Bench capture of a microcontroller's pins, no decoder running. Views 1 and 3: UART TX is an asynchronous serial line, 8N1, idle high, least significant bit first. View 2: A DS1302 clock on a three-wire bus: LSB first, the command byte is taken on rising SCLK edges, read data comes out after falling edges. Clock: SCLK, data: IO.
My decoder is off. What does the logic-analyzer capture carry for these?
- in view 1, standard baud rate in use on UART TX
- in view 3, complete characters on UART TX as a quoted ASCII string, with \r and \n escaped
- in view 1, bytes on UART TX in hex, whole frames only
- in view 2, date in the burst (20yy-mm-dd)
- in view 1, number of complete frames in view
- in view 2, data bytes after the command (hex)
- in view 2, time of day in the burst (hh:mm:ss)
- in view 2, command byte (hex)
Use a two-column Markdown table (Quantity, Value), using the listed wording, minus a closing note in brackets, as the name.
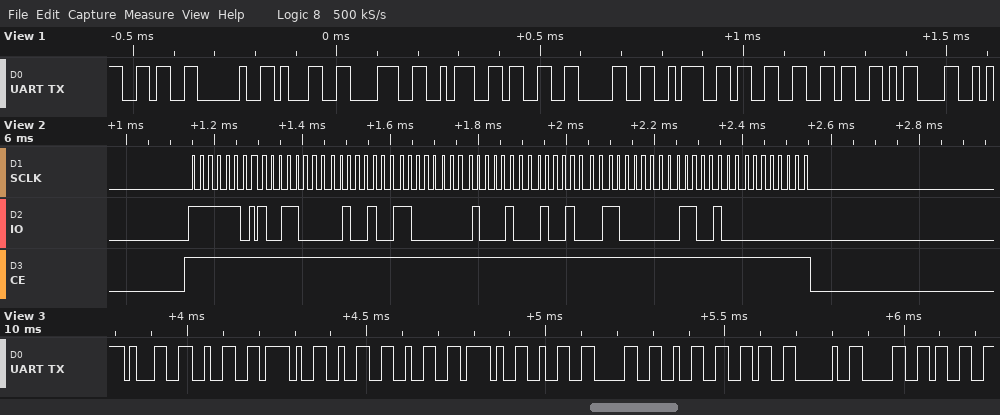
| Quantity | Value |
|---|---|
| in view 1, standard baud rate in use on UART TX | 57600 baud |
| in view 3, complete characters on UART TX as a quoted ASCII string, with \r and \n escaped | "12/22/2026 03" |
| in view 1, bytes on UART TX in hex, whole frames only | 36 20 31 38 3A 33 30 3A 33 36 0D |
| in view 2, date in the burst | 2026-12-22 |
| in view 1, number of complete frames in view | 11 |
| in view 2, data bytes after the command | 19 24 03 22 12 03 26 00 |
| in view 2, time of day in the burst | 03:24:19 |
| in view 2, command byte | 0xBF |
